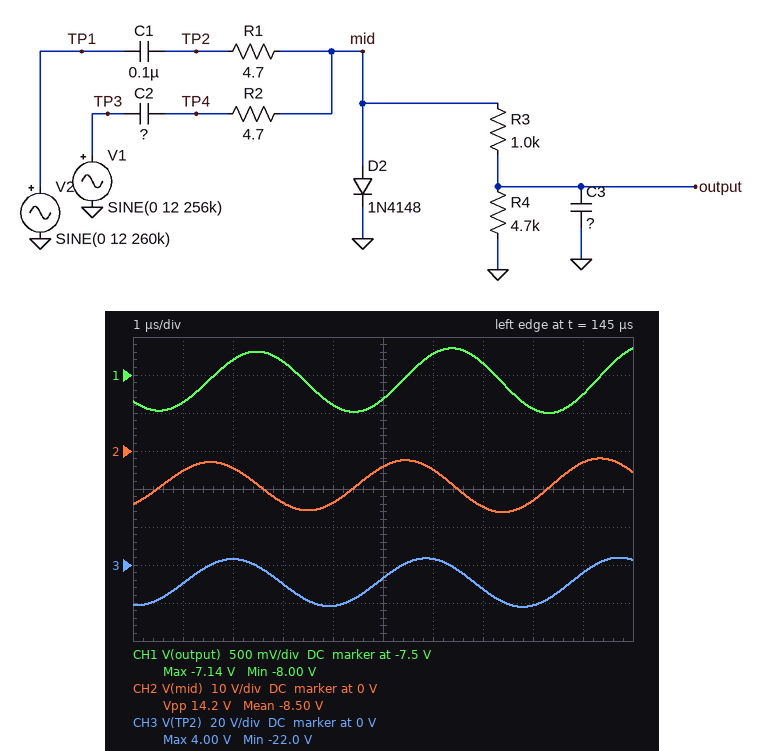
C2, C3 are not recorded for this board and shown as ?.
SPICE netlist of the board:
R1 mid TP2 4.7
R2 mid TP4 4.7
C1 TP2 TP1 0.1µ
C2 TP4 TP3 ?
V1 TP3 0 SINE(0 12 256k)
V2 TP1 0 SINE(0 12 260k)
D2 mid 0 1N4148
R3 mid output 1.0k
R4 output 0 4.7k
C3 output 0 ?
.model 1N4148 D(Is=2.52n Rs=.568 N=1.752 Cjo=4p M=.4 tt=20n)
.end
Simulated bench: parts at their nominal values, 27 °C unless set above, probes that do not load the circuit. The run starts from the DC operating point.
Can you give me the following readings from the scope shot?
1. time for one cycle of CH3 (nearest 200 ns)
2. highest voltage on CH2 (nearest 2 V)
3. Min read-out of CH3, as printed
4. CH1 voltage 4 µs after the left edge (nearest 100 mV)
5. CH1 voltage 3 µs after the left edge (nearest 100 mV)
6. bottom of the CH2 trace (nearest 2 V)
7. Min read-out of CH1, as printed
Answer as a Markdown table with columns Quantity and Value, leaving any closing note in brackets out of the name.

| Quantity | Value |
|---|---|
| time for one cycle of CH3 | 3.8 µs |
| highest voltage on CH2 | -2 V |
| Min read-out of CH3, as printed | -22.0 V |
| CH1 voltage 4 µs after the left edge | -7.9 V |
| CH1 voltage 3 µs after the left edge | -7.3 V |
| bottom of the CH2 trace | -16 V |
| Min read-out of CH1, as printed | -8.00 V |
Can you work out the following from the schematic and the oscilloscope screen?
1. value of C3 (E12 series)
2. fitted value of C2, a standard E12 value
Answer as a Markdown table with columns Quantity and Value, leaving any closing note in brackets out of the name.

| Quantity | Value |
|---|---|
| value of C3 | 10 nF |
| fitted value of C2, a standard E12 value | 270 nF |
